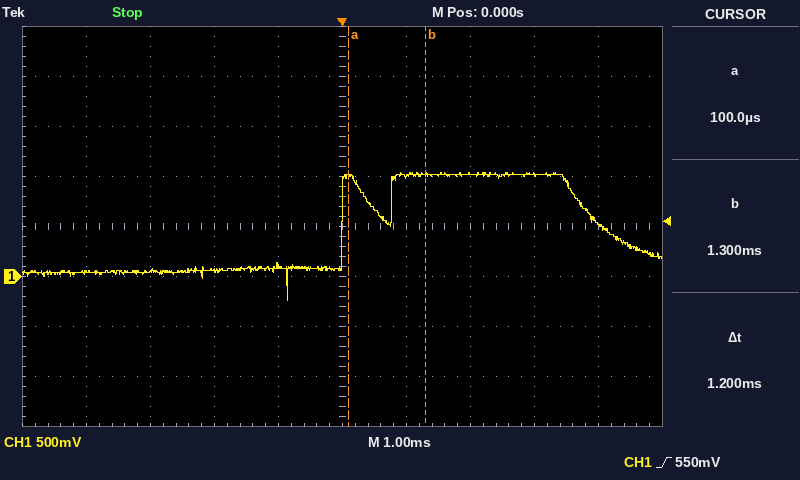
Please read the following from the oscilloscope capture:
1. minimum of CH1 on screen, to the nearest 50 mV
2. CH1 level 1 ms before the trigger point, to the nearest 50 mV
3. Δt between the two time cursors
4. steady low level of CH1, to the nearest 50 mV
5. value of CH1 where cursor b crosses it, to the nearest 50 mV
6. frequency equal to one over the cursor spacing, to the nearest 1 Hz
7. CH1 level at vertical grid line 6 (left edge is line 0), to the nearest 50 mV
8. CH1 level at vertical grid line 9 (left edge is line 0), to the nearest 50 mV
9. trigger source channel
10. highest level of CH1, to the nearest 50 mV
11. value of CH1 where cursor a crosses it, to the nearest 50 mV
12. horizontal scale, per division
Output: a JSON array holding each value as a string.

["-250 mV", "100 mV", "1.2 ms", "50 mV", "1.00 V", "833 Hz", "1.00 V", "550 mV", "CH1", "1.05 V", "1.00 V", "1 ms"]
